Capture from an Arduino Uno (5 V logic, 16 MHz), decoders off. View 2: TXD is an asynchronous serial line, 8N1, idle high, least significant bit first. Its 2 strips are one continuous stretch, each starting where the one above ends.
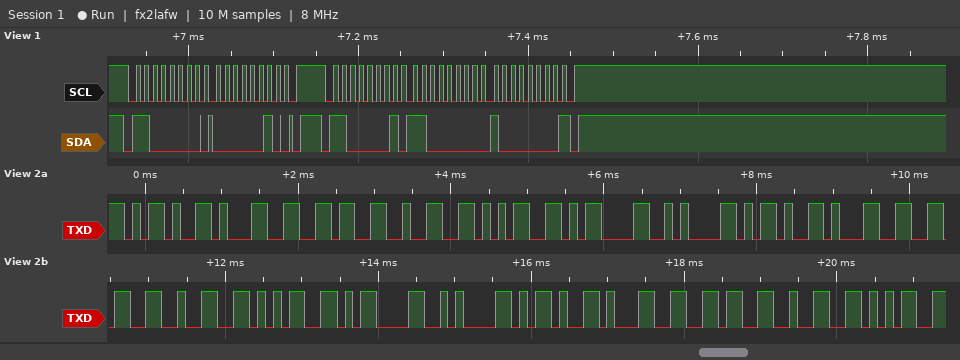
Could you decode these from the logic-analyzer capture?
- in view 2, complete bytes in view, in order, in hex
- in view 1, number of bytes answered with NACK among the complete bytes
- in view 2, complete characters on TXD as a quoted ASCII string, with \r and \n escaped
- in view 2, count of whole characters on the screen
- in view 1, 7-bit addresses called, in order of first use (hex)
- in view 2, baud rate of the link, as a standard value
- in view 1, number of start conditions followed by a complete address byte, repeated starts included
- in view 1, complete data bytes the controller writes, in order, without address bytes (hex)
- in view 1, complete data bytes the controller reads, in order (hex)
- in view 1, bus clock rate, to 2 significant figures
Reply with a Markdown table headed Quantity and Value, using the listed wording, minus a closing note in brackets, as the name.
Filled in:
| Quantity | Value |
|---|---|
| in view 2, complete bytes in view, in order, in hex | 2D 31 36 32 35 0D 0A 2D 31 36 32 35 0D 0A 2D 31 36 32 35 |
| in view 1, number of bytes answered with NACK among the complete bytes | 1 |
| in view 2, complete characters on TXD as a quoted ASCII string, with \r and \n escaped | "-1625\r\n-1625\r\n-1625" |
| in view 2, count of whole characters on the screen | 19 |
| in view 1, 7-bit addresses called, in order of first use | 0x60 |
| in view 2, baud rate of the link, as a standard value | 9600 baud |
| in view 1, number of start conditions followed by a complete address byte, repeated starts included | 2 |
| in view 1, complete data bytes the controller writes, in order, without address bytes | 02 |
| in view 1, complete data bytes the controller reads, in order | C0 80 |
| in view 1, bus clock rate, to 2 significant figures | 100 kHz |
